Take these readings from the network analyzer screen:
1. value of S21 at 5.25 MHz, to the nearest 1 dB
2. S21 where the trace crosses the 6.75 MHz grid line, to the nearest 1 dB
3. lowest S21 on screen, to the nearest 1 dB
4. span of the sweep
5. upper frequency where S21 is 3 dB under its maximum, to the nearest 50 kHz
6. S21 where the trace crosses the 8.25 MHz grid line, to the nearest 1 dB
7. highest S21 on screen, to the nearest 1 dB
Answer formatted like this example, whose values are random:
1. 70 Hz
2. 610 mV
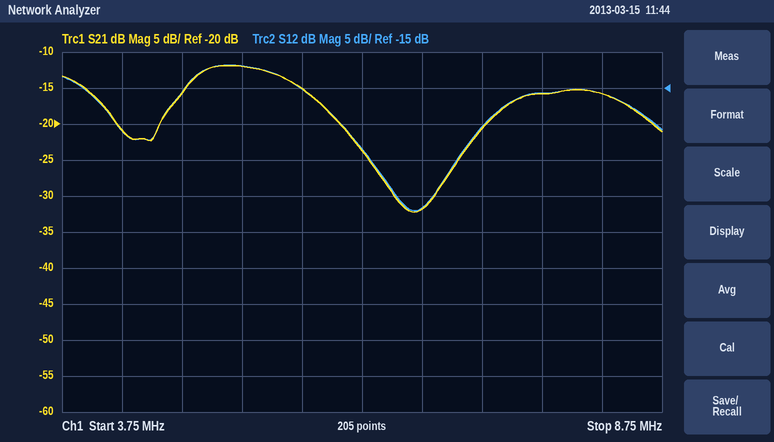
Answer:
1. -12 dB
2. -32 dB
3. -32 dB
4. 5 MHz
5. 5.75 MHz
6. -16 dB
7. -12 dB
